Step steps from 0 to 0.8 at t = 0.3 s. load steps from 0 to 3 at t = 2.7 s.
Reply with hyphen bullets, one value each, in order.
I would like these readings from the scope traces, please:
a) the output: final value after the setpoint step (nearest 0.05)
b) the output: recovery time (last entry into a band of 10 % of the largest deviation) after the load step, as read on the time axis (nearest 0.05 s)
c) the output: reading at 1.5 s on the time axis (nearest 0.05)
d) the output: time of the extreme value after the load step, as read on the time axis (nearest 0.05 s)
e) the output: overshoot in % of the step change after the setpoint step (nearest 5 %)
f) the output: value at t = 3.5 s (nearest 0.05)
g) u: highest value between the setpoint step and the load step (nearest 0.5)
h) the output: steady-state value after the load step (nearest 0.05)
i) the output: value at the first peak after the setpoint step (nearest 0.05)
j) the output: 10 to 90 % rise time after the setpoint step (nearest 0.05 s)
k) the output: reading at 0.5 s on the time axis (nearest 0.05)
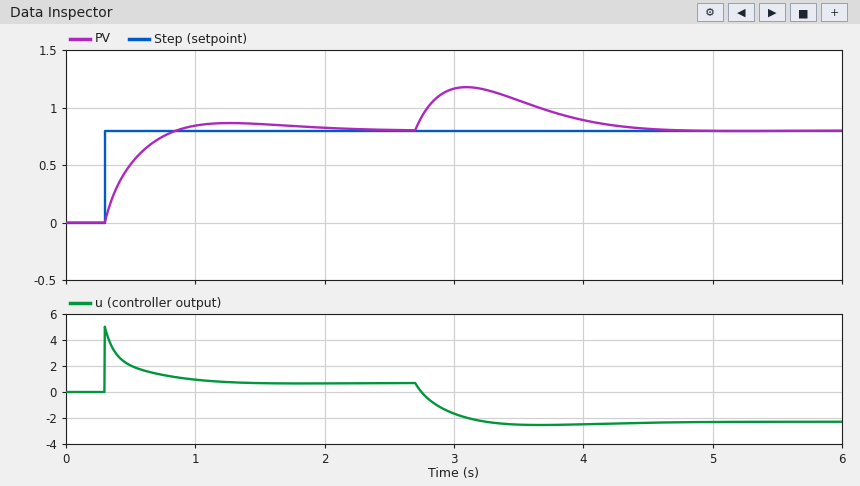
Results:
- 0.80
- 4.30 s
- 0.85
- 3.10 s
- 10 %
- 1.05
- 5.0
- 0.80
- 0.85
- 0.40 s
- 0.50
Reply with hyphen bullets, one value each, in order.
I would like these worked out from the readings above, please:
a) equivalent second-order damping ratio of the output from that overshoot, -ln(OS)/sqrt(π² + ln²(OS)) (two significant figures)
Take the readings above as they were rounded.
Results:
- 0.59
